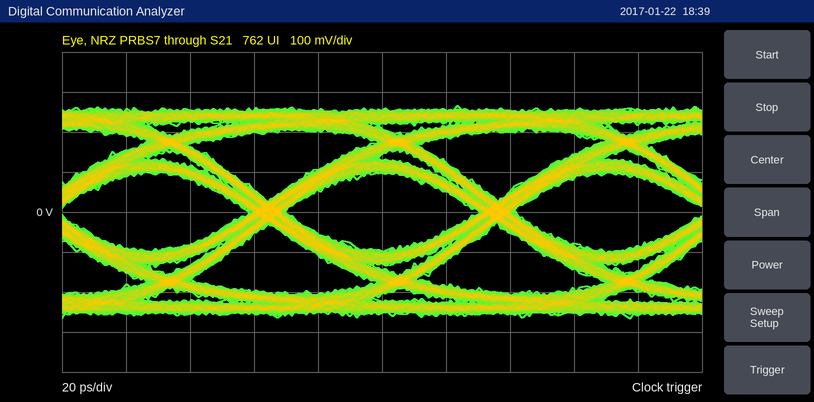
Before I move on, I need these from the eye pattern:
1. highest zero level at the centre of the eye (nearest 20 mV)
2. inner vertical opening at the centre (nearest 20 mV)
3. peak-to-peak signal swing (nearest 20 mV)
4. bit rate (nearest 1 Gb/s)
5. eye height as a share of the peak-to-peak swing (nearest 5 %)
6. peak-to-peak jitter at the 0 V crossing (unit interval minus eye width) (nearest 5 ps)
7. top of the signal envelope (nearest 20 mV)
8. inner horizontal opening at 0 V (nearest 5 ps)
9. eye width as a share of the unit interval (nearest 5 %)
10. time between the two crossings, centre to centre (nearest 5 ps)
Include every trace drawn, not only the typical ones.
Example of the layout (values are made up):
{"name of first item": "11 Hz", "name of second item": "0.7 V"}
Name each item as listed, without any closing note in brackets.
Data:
{"highest zero level at the centre of the eye": "-100 mV", "inner vertical opening at the centre": "200 mV", "peak-to-peak signal swing": "540 mV", "bit rate": "14 Gb/s", "eye height as a share of the peak-to-peak swing": "35 %", "peak-to-peak jitter at the 0 V crossing (unit interval minus eye width)": "10 ps", "top of the signal envelope": "260 mV", "inner horizontal opening at 0 V": "60 ps", "eye width as a share of the unit interval": "85 %", "time between the two crossings, centre to centre": "70 ps"}
